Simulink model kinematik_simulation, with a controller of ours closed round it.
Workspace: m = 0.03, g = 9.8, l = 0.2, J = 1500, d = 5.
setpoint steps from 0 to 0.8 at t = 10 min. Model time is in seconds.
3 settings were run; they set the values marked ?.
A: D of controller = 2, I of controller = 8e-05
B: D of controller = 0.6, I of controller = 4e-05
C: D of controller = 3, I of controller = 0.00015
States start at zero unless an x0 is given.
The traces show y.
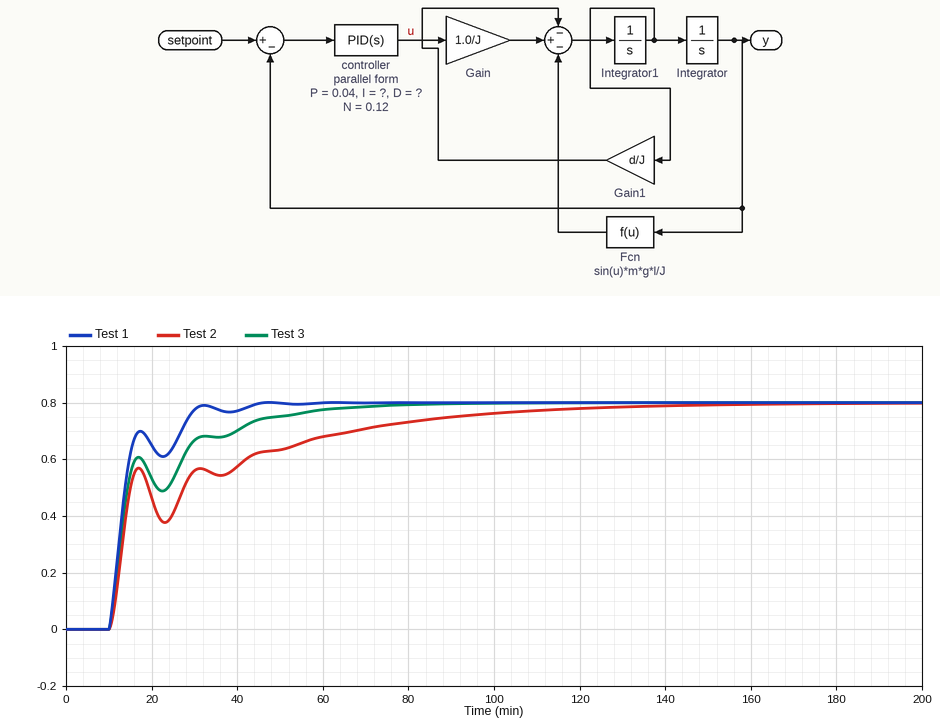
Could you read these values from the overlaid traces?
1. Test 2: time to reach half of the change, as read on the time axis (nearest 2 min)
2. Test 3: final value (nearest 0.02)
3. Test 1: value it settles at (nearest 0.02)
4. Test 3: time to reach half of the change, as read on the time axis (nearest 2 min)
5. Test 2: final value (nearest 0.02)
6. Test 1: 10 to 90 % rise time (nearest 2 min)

14 min
0.80
0.80
14 min
0.80
16 min
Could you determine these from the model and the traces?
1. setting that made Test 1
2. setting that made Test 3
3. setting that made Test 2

C
A
B
